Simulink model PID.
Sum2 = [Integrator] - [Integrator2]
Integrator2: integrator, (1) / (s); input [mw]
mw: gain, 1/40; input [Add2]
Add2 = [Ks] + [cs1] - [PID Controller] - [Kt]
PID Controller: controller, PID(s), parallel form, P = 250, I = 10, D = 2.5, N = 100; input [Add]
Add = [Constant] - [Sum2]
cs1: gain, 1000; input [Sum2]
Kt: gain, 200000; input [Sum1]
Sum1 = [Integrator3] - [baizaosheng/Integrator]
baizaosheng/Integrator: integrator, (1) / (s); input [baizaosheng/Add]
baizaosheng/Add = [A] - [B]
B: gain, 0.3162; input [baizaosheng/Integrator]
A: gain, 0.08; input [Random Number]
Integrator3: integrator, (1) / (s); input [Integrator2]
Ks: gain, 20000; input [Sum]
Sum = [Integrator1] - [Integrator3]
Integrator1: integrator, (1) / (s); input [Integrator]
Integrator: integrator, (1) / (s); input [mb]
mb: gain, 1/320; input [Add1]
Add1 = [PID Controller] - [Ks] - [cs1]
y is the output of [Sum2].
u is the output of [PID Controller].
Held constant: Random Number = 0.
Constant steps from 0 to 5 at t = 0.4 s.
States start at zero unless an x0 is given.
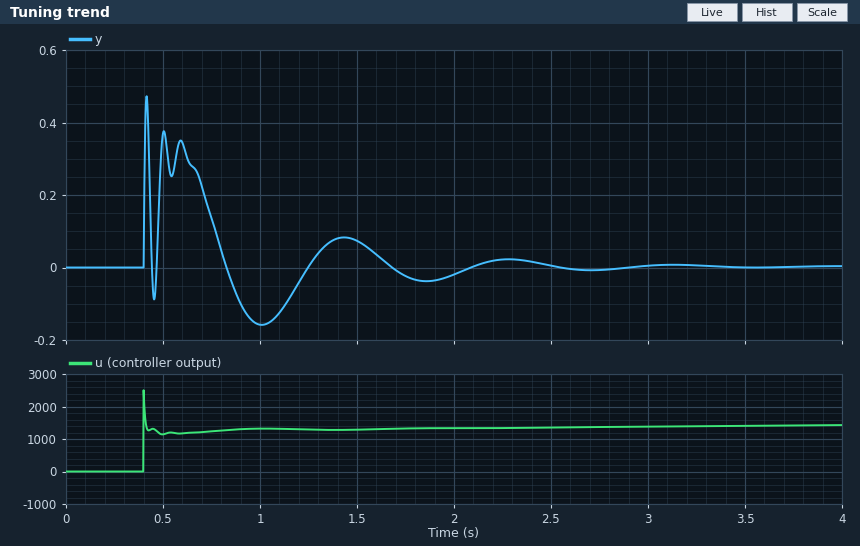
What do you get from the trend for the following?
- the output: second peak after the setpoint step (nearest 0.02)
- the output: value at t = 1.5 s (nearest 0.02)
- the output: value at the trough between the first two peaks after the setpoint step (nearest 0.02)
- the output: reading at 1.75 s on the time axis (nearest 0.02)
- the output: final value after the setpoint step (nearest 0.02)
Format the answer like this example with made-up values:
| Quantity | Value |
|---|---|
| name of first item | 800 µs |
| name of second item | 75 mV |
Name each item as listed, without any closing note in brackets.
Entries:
| Quantity | Value |
|---|---|
| the output: second peak after the setpoint step | 0.38 |
| the output: value at t = 1.5 s | 0.08 |
| the output: value at the trough between the first two peaks after the setpoint step | -0.08 |
| the output: reading at 1.75 s on the time axis | -0.02 |
| the output: final value after the setpoint step | 0.00 |
